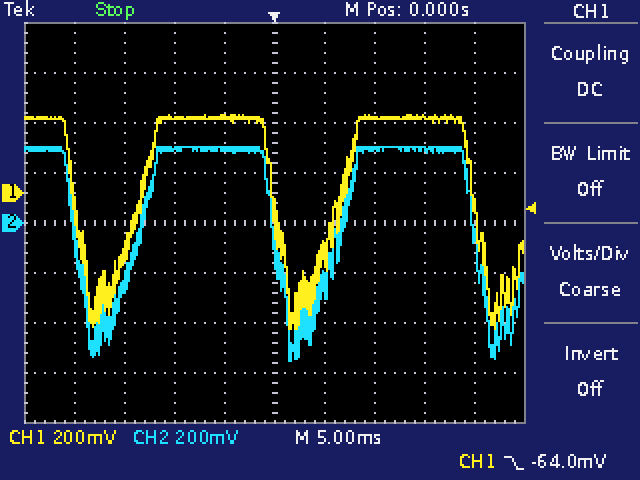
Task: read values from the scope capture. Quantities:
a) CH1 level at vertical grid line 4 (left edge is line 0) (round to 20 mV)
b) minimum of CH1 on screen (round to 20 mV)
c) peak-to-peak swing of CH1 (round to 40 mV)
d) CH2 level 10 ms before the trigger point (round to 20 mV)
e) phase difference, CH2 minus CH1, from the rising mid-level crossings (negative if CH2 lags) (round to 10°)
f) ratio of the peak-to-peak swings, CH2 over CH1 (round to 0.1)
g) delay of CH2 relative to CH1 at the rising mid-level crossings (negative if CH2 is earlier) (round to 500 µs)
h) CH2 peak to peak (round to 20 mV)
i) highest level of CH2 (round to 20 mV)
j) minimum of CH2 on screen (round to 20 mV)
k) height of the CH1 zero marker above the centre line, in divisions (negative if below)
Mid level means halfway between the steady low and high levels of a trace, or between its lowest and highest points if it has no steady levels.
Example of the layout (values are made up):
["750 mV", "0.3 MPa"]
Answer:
["300 mV", "-540 mV", "840 mV", "300 mV", "0°", "1.0", "0.0 ms", "860 mV", "300 mV", "-560 mV", "+0.6 div"]
